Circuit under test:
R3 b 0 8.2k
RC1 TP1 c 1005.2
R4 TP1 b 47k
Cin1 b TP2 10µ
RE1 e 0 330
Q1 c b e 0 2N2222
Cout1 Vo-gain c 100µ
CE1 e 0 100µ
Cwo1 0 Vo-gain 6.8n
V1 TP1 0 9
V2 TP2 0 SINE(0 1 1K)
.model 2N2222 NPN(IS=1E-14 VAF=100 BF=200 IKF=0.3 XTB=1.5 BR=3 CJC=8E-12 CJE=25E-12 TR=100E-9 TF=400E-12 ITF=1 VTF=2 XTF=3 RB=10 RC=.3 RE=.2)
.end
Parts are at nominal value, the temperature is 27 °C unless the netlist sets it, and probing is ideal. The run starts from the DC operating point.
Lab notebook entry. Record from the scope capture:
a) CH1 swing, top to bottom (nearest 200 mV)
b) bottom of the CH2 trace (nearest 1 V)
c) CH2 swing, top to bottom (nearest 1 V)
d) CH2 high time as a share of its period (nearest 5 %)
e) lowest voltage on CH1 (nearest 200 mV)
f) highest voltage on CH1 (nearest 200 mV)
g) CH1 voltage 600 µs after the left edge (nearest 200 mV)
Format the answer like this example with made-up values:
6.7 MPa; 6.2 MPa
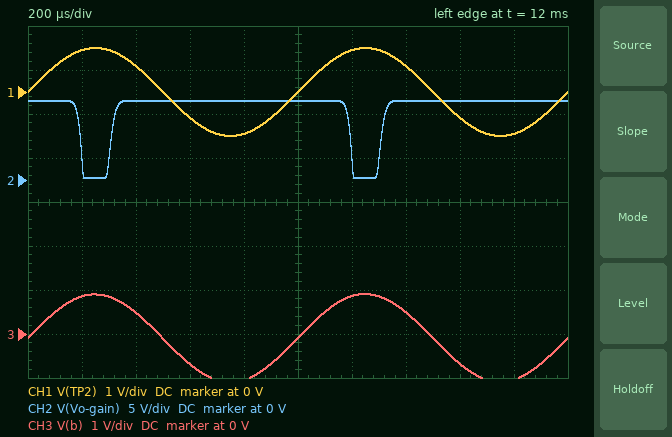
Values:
2.0 V; 0 V; 9 V; 90 %; -1.0 V; 1.0 V; -600 mV
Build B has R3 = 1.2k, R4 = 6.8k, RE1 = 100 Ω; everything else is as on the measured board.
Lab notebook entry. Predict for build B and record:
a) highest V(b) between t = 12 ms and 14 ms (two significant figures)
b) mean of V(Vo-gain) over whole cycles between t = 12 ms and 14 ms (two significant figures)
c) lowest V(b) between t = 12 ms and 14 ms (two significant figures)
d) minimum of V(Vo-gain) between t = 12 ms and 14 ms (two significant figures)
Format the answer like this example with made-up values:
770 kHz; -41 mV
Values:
1.1 V; 7.3 V; -910 mV; 220 mV
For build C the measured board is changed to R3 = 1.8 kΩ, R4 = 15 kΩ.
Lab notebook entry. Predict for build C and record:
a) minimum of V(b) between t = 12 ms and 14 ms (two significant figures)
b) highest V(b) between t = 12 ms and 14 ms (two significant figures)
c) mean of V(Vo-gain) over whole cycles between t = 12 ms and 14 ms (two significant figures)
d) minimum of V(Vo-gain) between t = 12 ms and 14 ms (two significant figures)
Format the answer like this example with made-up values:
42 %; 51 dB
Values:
-980 mV; 1.0 V; 7.6 V; 230 mV
